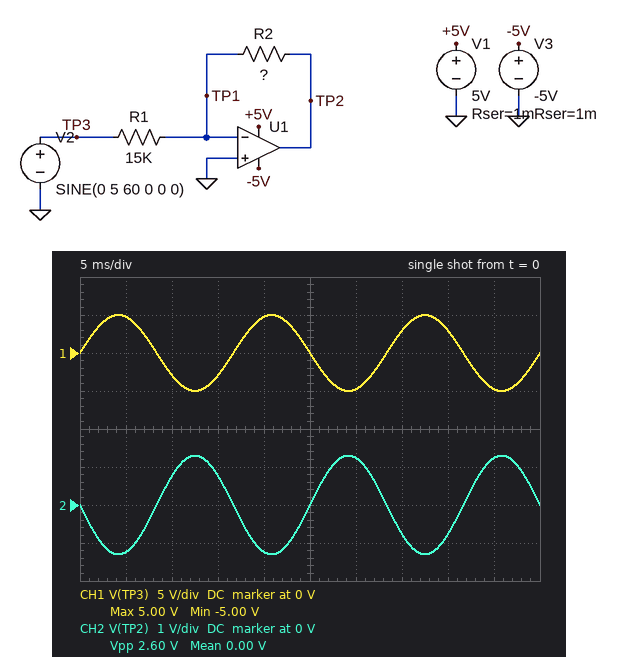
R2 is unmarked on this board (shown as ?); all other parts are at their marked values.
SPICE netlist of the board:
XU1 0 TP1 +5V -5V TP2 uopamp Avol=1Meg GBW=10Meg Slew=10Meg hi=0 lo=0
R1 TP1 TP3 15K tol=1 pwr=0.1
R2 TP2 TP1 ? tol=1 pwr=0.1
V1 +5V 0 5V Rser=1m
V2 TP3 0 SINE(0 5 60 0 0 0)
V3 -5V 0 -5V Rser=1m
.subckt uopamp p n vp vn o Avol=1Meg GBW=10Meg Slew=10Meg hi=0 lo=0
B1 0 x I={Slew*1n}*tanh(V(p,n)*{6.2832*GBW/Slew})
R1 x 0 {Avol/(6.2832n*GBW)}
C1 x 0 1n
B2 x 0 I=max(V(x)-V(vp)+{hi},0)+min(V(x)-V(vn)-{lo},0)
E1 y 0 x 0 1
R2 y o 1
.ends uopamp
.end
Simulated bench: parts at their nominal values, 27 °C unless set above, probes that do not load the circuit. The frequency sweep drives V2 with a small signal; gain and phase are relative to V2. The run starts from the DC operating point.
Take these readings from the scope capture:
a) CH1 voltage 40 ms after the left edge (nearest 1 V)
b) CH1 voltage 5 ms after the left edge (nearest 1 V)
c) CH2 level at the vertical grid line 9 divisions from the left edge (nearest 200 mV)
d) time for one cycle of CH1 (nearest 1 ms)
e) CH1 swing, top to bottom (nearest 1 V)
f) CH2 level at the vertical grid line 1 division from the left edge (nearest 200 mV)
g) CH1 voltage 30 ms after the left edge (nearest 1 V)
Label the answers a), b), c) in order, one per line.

a) 3 V
b) 5 V
c) 1.2 V
d) 17 ms
e) 10 V
f) -1.2 V
g) -5 V
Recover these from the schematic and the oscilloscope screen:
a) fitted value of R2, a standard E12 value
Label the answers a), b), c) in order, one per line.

a) 3.9 kΩ
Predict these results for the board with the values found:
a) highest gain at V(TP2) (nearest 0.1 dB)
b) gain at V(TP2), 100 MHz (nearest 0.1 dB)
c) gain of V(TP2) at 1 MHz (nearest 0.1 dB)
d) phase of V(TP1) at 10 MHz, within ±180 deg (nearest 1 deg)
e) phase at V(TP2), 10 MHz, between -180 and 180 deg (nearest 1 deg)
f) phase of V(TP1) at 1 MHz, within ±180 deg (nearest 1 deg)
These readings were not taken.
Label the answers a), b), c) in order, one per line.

a) -11.7 dB
b) -33.7 dB
c) -11.8 dB
d) 38 deg
e) 128 deg
f) 83 deg
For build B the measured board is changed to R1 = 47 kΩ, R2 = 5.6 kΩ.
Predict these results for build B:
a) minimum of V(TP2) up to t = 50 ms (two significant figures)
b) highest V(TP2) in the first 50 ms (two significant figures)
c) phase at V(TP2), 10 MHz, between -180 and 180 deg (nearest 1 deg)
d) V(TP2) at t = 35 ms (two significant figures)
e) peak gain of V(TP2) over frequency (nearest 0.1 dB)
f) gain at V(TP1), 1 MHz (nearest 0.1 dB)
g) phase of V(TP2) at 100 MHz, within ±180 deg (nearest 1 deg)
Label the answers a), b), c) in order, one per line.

a) -600 mV
b) 600 mV
c) 132 deg
d) -350 mV
e) -18.5 dB
f) -38.5 dB
g) 95 deg
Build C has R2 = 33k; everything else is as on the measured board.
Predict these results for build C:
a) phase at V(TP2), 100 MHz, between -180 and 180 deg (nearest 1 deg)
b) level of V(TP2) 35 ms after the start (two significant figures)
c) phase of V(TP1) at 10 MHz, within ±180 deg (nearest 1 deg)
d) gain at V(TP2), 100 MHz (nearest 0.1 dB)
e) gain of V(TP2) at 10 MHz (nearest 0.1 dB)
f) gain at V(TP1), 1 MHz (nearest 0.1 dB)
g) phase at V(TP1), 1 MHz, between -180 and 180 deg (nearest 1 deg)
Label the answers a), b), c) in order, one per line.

a) 92 deg
b) -5.0 V
c) 17 deg
d) -23.3 dB
e) -3.7 dB
f) -13.6 dB
g) 72 deg
